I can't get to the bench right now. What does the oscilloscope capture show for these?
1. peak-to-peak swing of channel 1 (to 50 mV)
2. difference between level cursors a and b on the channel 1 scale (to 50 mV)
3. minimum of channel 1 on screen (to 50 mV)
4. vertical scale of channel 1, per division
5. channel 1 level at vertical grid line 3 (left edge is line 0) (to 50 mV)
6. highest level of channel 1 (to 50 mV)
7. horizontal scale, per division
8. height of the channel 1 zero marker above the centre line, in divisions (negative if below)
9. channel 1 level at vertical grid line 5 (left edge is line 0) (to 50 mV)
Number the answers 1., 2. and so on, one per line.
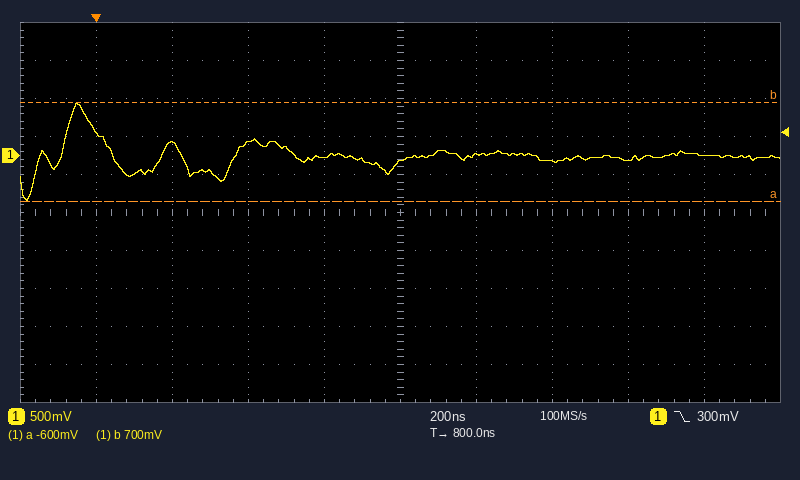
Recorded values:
1. 1.30 V
2. 1.30 V
3. -600 mV
4. 500 mV
5. 150 mV
6. 700 mV
7. 200 ns
8. +1.5 div
9. -100 mV
